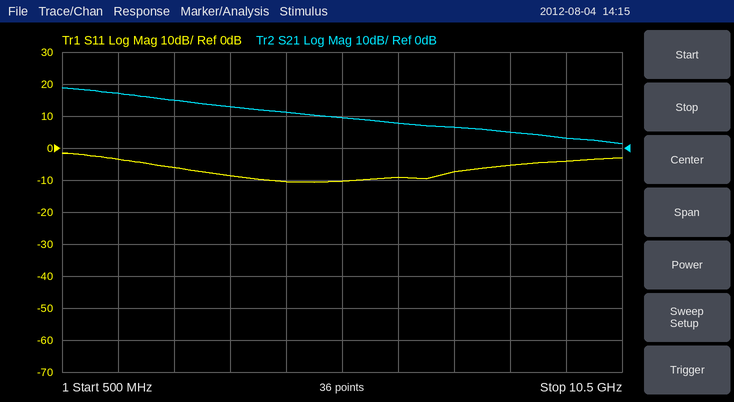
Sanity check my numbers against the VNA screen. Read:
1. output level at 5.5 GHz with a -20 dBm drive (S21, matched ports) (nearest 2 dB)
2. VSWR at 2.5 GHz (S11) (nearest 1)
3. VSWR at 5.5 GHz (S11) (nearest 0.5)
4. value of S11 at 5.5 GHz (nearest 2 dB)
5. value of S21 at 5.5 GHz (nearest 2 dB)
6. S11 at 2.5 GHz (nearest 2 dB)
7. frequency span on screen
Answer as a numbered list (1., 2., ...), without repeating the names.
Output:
1. -10 dBm
2. 3
3. 2.0
4. -10 dB
5. 10 dB
6. -6 dB
7. 10 GHz
